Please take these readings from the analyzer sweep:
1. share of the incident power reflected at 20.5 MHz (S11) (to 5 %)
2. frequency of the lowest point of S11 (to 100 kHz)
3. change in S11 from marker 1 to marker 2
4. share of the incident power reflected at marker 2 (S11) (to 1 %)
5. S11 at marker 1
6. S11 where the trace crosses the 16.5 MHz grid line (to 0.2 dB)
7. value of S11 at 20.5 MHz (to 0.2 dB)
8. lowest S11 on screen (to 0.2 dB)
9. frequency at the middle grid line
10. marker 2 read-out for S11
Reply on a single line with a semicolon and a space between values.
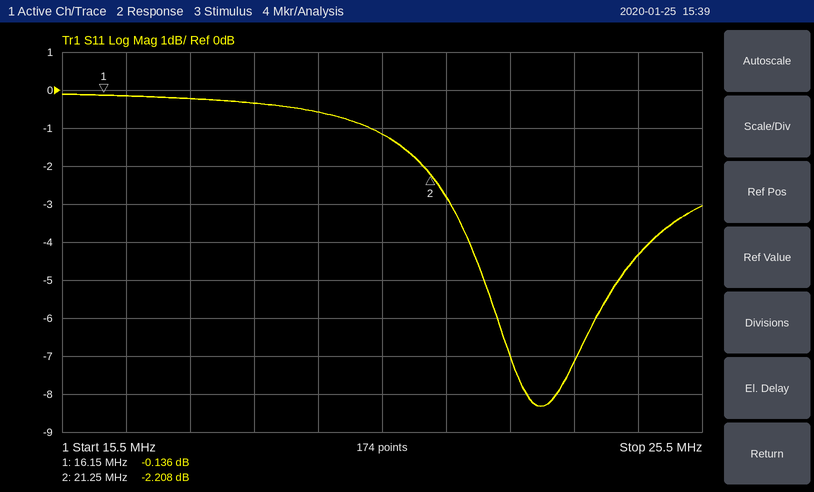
75 %; 23.0 MHz; -2.072 dB; 60 %; -0.136 dB; -0.2 dB; -1.2 dB; -8.4 dB; 20.5 MHz; -2.208 dB
